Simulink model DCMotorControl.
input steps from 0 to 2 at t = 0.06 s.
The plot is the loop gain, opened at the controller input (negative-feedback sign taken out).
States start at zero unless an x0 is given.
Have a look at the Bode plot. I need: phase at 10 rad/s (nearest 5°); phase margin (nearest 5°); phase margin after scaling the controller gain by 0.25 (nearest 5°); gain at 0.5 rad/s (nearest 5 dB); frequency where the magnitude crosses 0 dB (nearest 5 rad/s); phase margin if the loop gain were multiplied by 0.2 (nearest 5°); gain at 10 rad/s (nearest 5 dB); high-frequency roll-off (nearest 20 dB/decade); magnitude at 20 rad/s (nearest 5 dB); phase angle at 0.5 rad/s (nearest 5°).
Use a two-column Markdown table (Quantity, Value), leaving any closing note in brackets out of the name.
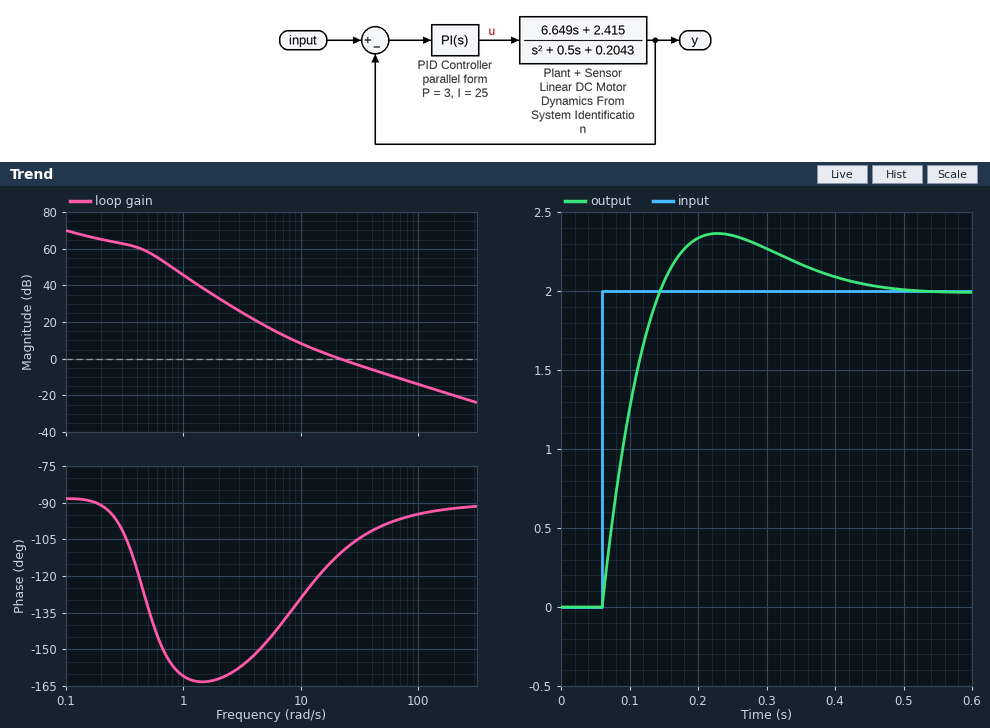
| Quantity | Value |
|---|---|
| phase at 10 rad/s | -130° |
| phase margin | 70° |
| phase margin after scaling the controller gain by 0.25 | 45° |
| gain at 0.5 rad/s | 60 dB |
| frequency where the magnitude crosses 0 dB | 20 rad/s |
| phase margin if the loop gain were multiplied by 0.2 | 40° |
| gain at 10 rad/s | 10 dB |
| high-frequency roll-off | -20 dB/decade |
| magnitude at 20 rad/s | 0 dB |
| phase angle at 0.5 rad/s | -135° |
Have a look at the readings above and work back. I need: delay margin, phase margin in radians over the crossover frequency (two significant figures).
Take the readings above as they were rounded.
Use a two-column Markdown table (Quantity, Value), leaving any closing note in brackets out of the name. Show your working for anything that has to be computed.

| Quantity | Value |
|---|---|
| delay margin, phase margin in radians over the crossover frequency | 70 × π / 180 / 20 = 0.061 s |
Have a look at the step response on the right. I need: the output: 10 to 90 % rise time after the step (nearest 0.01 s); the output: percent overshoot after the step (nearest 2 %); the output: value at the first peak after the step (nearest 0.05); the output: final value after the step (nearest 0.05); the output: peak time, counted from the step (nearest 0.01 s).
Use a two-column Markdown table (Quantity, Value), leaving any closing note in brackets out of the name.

| Quantity | Value |
|---|---|
| the output: 10 to 90 % rise time after the step | 0.06 s |
| the output: percent overshoot after the step | 18 % |
| the output: value at the first peak after the step | 2.35 |
| the output: final value after the step | 2.00 |
| the output: peak time, counted from the step | 0.17 s |
